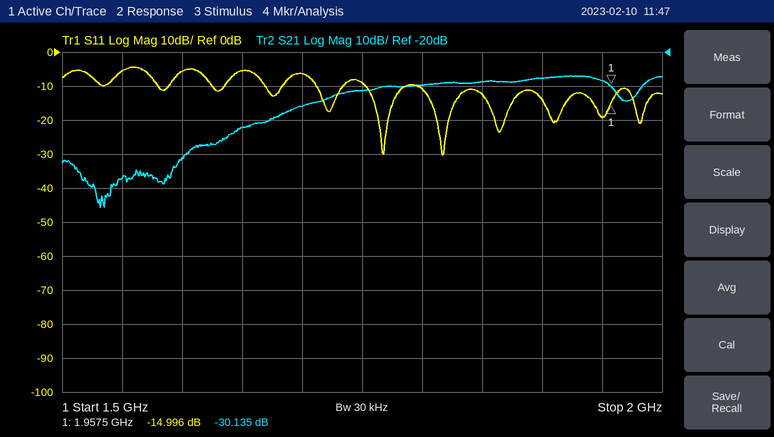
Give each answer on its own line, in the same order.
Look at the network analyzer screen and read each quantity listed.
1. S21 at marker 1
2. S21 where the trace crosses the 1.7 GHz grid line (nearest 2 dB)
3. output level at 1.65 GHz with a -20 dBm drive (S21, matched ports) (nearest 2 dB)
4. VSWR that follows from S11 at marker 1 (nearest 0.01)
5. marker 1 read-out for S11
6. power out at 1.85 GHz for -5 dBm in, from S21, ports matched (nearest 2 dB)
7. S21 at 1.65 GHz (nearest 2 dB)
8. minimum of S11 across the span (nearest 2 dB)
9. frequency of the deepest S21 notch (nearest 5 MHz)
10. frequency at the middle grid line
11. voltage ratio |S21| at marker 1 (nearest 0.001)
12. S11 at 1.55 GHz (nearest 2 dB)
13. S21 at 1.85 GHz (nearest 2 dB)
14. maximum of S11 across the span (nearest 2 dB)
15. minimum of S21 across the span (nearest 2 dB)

-30.135 dB
-36 dB
-62 dBm
1.43
-14.996 dB
-34 dBm
-42 dB
-30 dB
1.530 GHz
1.75 GHz
0.031
-6 dB
-28 dB
-4 dB
-66 dB
